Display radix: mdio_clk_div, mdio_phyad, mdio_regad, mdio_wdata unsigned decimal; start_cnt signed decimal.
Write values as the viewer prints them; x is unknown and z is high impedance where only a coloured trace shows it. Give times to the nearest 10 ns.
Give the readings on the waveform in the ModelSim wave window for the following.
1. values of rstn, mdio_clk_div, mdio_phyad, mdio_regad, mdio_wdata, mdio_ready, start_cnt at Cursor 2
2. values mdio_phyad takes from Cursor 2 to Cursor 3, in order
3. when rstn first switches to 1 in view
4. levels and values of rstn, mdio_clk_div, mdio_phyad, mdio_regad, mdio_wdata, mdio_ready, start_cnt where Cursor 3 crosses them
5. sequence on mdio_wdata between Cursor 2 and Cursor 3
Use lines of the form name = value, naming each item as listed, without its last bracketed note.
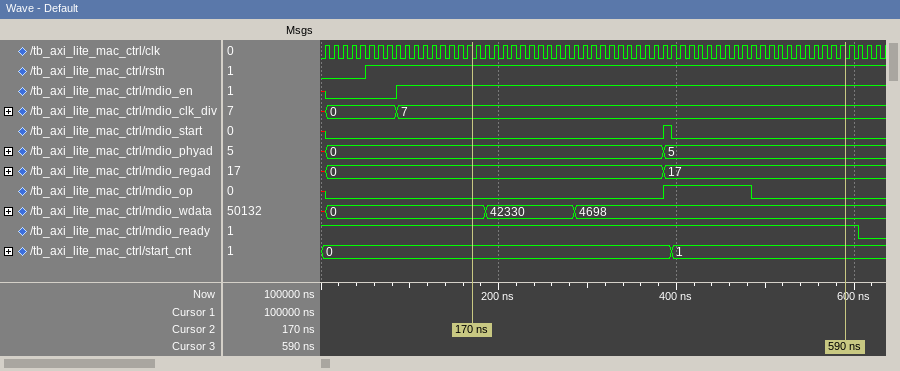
values of rstn, mdio_clk_div, mdio_phyad, mdio_regad, mdio_wdata, mdio_ready, start_cnt at Cursor 2 = rstn=1, mdio_clk_div=7, mdio_phyad=0, mdio_regad=0, mdio_wdata=0, mdio_ready=1, start_cnt=0
values mdio_phyad takes from Cursor 2 to Cursor 3, in order = 0, 5
when rstn first switches to 1 in view = 50 ns
levels and values of rstn, mdio_clk_div, mdio_phyad, mdio_regad, mdio_wdata, mdio_ready, start_cnt where Cursor 3 crosses them = rstn=1, mdio_clk_div=7, mdio_phyad=5, mdio_regad=17, mdio_wdata=4698, mdio_ready=1, start_cnt=1
sequence on mdio_wdata between Cursor 2 and Cursor 3 = 0, 42330, 4698
